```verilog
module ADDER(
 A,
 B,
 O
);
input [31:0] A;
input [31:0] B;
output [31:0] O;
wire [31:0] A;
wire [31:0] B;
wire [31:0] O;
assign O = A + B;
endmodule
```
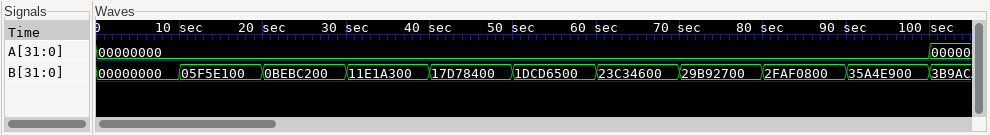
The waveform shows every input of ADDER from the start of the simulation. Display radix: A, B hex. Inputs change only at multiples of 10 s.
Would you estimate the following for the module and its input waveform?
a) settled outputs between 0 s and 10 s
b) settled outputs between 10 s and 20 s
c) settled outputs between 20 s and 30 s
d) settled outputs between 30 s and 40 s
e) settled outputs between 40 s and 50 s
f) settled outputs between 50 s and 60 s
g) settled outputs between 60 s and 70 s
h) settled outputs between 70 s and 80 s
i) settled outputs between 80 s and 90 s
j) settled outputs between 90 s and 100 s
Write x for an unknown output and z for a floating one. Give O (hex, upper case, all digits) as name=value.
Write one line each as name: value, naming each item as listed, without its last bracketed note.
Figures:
settled outputs between 0 s and 10 s: O=00000000
settled outputs between 10 s and 20 s: O=05F5E100
settled outputs between 20 s and 30 s: O=0BEBC200
settled outputs between 30 s and 40 s: O=11E1A300
settled outputs between 40 s and 50 s: O=17D78400
settled outputs between 50 s and 60 s: O=1DCD6500
settled outputs between 60 s and 70 s: O=23C34600
settled outputs between 70 s and 80 s: O=29B92700
settled outputs between 80 s and 90 s: O=2FAF0800
settled outputs between 90 s and 100 s: O=35A4E900
